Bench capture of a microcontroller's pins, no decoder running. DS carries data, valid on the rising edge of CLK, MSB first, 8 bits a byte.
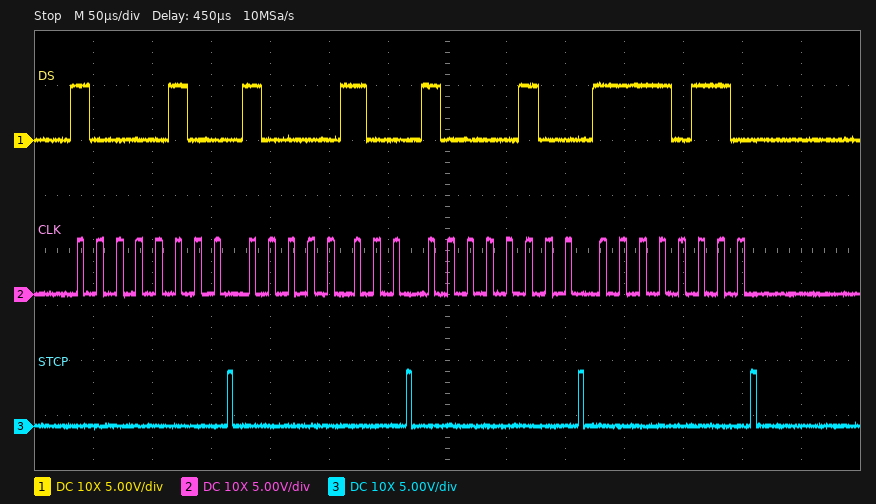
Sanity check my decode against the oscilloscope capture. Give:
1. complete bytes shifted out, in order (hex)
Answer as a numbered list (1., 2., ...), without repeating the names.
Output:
1. 84 84 84 F6
